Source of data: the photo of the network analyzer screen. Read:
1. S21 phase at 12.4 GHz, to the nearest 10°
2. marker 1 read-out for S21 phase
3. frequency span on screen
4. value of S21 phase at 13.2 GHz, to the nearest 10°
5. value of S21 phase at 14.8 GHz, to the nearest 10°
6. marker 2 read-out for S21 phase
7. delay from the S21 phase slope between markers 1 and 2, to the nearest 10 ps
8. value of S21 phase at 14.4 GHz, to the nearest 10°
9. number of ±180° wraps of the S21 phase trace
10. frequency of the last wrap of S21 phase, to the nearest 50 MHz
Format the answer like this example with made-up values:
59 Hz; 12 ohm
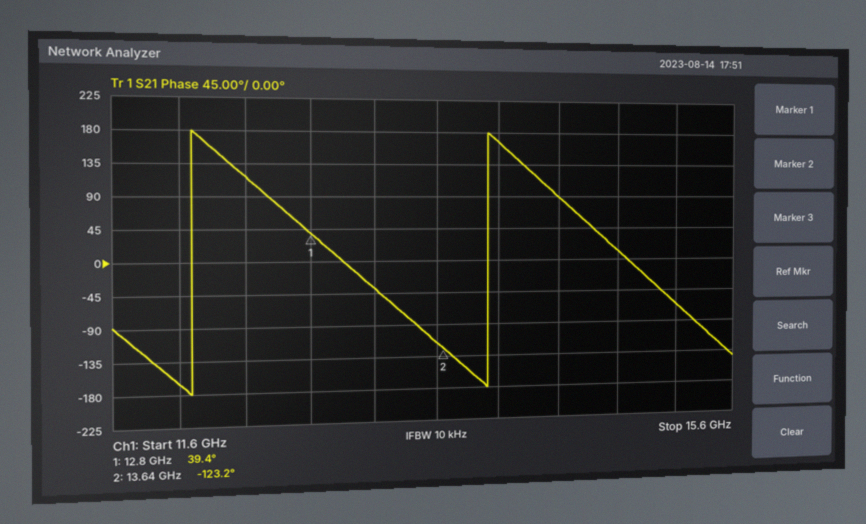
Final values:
120°; 39.4°; 4 GHz; -40°; 10°; -123.2°; 540 ps; 90°; 2; 13.95 GHz
